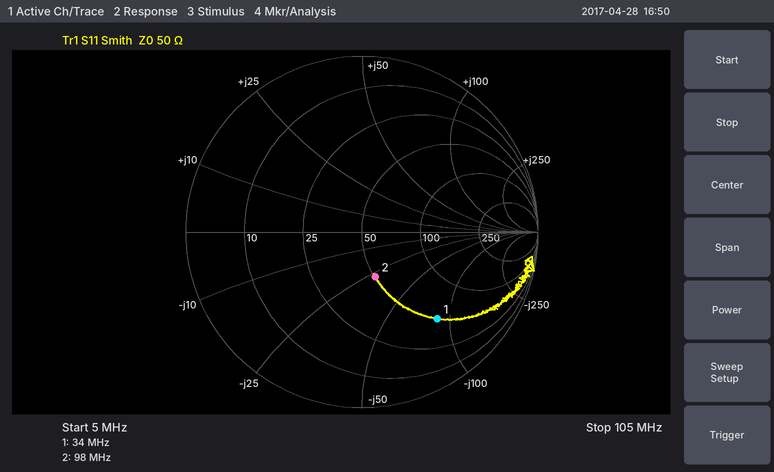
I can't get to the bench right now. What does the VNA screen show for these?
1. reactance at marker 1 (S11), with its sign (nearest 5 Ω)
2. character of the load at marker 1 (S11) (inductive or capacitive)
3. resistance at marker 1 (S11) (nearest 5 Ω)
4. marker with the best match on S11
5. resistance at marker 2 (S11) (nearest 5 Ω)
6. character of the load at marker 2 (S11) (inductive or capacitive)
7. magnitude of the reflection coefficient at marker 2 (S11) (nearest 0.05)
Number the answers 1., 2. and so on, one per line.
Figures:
1. -85 Ω
2. capacitive
3. 50 Ω
4. marker 2
5. 50 Ω
6. capacitive
7. 0.25
